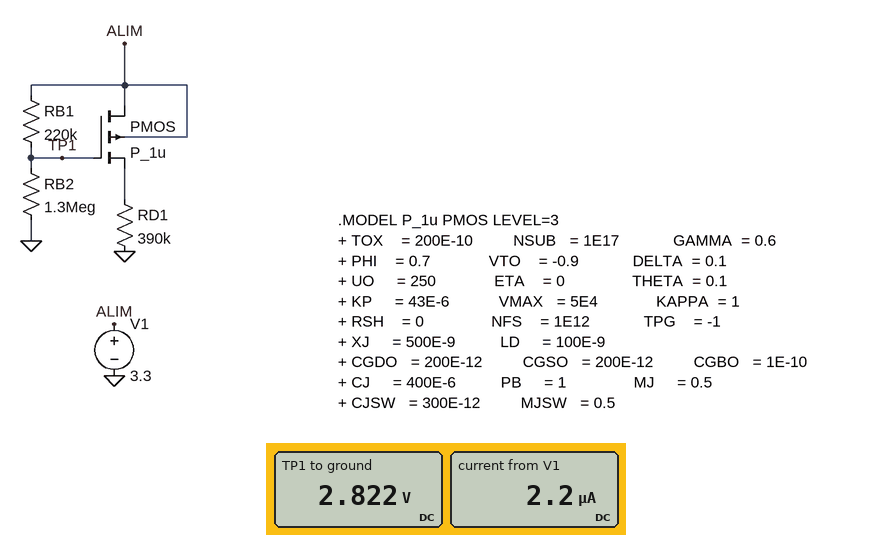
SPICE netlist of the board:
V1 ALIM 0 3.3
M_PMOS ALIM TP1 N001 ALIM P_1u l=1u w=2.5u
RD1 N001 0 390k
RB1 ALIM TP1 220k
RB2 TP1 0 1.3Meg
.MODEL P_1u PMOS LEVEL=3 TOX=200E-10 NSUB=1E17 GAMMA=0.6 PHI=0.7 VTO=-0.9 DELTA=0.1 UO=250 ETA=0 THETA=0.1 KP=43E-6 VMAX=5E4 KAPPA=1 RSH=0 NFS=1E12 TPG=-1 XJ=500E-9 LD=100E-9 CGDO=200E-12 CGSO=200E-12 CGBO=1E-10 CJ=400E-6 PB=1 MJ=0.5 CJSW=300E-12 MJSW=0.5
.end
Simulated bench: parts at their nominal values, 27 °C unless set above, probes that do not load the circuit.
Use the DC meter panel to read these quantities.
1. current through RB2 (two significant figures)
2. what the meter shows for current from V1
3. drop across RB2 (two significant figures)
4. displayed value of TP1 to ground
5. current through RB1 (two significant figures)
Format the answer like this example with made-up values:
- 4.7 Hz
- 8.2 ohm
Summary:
- 2.2 µA
- 2.2 µA
- 2.8 V
- 2.822 V
- 2.2 µA
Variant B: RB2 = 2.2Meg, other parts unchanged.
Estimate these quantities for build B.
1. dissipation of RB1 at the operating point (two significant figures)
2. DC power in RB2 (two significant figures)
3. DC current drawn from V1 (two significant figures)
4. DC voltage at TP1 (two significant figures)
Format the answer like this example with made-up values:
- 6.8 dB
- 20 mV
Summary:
- 410 nW
- 4.1 µW
- 1.4 µA
- 3.0 V
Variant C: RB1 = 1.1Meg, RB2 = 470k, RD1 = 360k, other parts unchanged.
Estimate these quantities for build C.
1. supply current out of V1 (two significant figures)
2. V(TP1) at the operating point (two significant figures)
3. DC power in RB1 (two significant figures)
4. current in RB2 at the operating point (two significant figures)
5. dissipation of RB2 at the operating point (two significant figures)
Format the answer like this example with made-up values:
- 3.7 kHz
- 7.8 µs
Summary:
- 11 µA
- 990 mV
- 4.9 µW
- 2.1 µA
- 2.1 µW
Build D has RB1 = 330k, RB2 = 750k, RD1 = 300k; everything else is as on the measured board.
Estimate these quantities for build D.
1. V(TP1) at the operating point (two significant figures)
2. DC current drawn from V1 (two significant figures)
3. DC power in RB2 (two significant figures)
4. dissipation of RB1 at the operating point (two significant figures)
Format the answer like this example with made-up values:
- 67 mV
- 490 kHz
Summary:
- 2.3 V
- 4.8 µA
- 7.0 µW
- 3.1 µW
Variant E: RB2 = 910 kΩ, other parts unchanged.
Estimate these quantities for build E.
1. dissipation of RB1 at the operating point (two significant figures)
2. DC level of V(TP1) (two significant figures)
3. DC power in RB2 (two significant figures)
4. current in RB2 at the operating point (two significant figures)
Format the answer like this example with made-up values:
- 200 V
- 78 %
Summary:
- 1.9 µW
- 2.7 V
- 7.8 µW
- 2.9 µA
